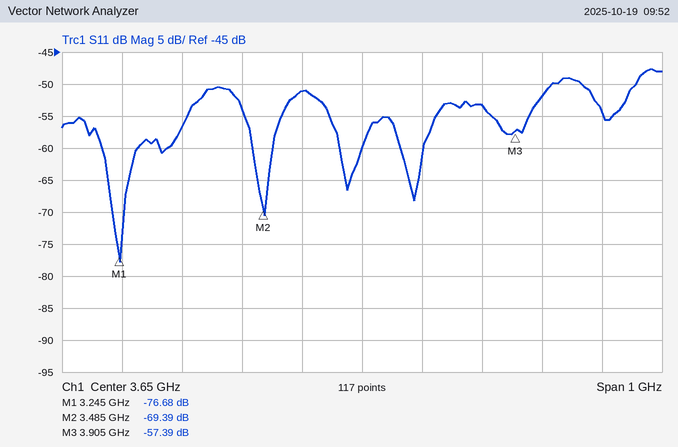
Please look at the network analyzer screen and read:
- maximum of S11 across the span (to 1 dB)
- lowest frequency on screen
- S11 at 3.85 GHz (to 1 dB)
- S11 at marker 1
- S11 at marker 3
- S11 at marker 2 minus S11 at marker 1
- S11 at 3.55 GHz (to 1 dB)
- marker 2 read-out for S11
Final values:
-48 dB
3.15 GHz
-53 dB
-76.68 dB
-57.39 dB
7.29 dB
-51 dB
-69.39 dB
